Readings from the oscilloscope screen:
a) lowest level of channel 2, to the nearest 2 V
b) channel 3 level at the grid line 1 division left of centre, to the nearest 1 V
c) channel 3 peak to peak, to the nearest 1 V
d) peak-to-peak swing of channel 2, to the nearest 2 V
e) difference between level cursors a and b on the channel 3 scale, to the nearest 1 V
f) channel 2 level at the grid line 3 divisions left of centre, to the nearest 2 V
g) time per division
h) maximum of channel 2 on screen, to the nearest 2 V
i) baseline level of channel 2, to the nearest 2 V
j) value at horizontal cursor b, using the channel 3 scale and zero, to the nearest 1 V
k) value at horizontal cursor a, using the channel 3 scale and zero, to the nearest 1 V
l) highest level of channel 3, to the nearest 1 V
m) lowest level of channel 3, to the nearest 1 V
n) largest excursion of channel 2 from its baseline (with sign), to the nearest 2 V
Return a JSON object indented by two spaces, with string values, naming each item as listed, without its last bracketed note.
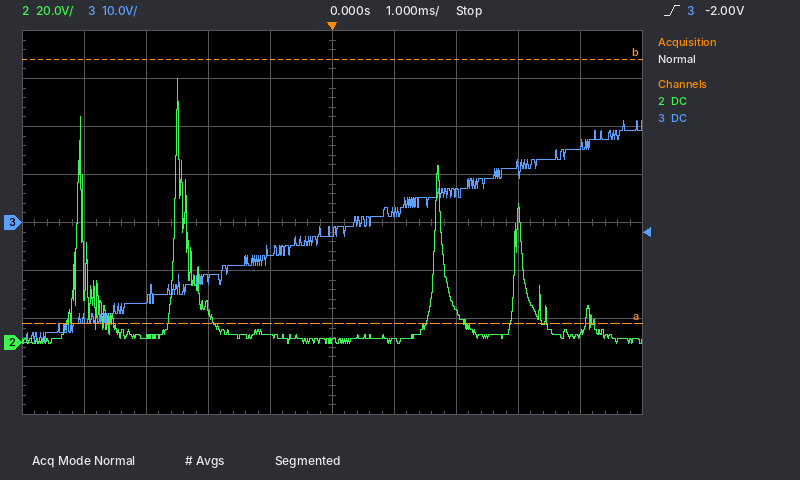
{
  "lowest level of channel 2, to the nearest 2 V": "0 V",
  "channel 3 level at the grid line 1 division left of centre, to the nearest 1 V": "-6 V",
  "channel 3 peak to peak, to the nearest 1 V": "46 V",
  "peak-to-peak swing of channel 2, to the nearest 2 V": "110 V",
  "difference between level cursors a and b on the channel 3 scale, to the nearest 1 V": "55 V",
  "channel 2 level at the grid line 3 divisions left of centre, to the nearest 2 V": "2 V",
  "time per division": "1 ms",
  "maximum of channel 2 on screen, to the nearest 2 V": "110 V",
  "baseline level of channel 2, to the nearest 2 V": "2 V",
  "value at horizontal cursor b, using the channel 3 scale and zero, to the nearest 1 V": "34 V",
  "value at horizontal cursor a, using the channel 3 scale and zero, to the nearest 1 V": "-21 V",
  "highest level of channel 3, to the nearest 1 V": "21 V",
  "lowest level of channel 3, to the nearest 1 V": "-25 V",
  "largest excursion of channel 2 from its baseline (with sign), to the nearest 2 V": "+108 V"
}
